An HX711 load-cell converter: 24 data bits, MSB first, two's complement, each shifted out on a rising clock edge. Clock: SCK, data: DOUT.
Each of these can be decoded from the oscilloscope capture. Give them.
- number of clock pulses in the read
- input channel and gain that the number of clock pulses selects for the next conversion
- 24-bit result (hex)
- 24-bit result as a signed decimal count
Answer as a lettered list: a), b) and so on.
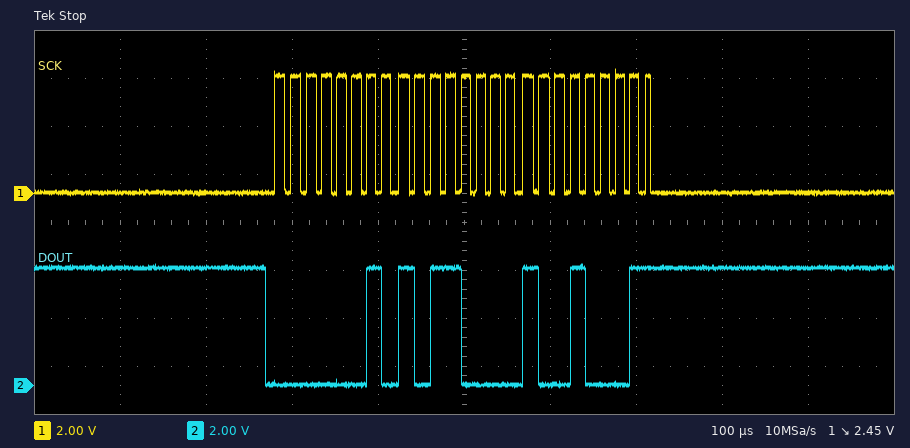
a) 25
b) channel A, gain 128
c) 0x02B091
d) 176273
